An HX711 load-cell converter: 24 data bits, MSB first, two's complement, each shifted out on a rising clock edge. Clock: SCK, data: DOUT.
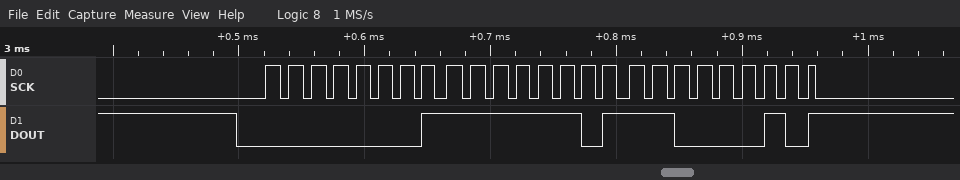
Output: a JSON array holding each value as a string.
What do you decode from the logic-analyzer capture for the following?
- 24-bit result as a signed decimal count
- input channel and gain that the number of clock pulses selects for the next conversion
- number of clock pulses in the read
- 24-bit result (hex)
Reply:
["130498", "channel A, gain 128", "25", "0x01FDC2"]
